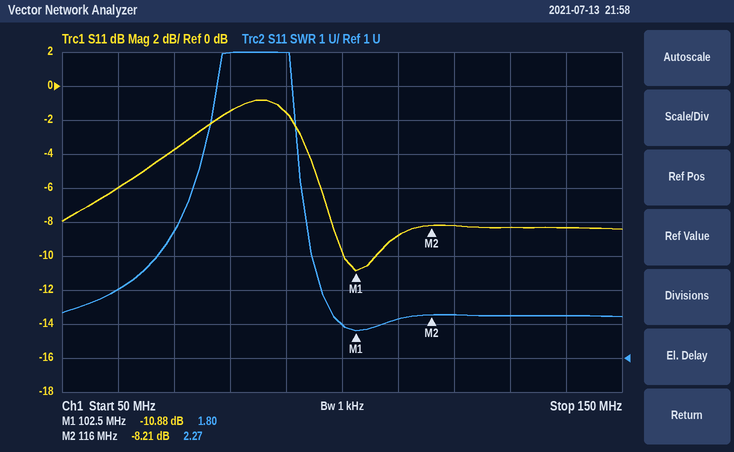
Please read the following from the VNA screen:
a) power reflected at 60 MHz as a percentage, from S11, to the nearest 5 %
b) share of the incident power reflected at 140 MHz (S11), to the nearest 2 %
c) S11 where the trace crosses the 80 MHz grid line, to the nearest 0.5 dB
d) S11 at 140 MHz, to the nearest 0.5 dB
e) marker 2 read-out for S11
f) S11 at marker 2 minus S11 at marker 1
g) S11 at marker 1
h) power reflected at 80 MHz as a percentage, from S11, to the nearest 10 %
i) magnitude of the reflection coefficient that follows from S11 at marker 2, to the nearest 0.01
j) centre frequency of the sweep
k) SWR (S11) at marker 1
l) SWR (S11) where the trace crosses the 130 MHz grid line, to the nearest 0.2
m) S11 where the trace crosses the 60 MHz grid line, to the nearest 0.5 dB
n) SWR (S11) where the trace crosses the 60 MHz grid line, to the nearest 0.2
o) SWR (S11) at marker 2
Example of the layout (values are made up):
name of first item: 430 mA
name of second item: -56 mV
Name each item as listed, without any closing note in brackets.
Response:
power reflected at 60 MHz as a percentage, from S11, to the nearest 5 %: 25 %
share of the incident power reflected at 140 MHz (S11), to the nearest 2 %: 14 %
S11 where the trace crosses the 80 MHz grid line, to the nearest 0.5 dB: -1.5 dB
S11 at 140 MHz, to the nearest 0.5 dB: -8.5 dB
marker 2 read-out for S11: -8.21 dB
S11 at marker 2 minus S11 at marker 1: 2.67 dB
S11 at marker 1: -10.88 dB
power reflected at 80 MHz as a percentage, from S11, to the nearest 10 %: 70 %
magnitude of the reflection coefficient that follows from S11 at marker 2, to the nearest 0.01: 0.39
centre frequency of the sweep: 100 MHz
SWR (S11) at marker 1: 1.80
SWR (S11) where the trace crosses the 130 MHz grid line, to the nearest 0.2: 2.2
S11 where the trace crosses the 60 MHz grid line, to the nearest 0.5 dB: -6.0 dB
SWR (S11) where the trace crosses the 60 MHz grid line, to the nearest 0.2: 3.0
SWR (S11) at marker 2: 2.27
